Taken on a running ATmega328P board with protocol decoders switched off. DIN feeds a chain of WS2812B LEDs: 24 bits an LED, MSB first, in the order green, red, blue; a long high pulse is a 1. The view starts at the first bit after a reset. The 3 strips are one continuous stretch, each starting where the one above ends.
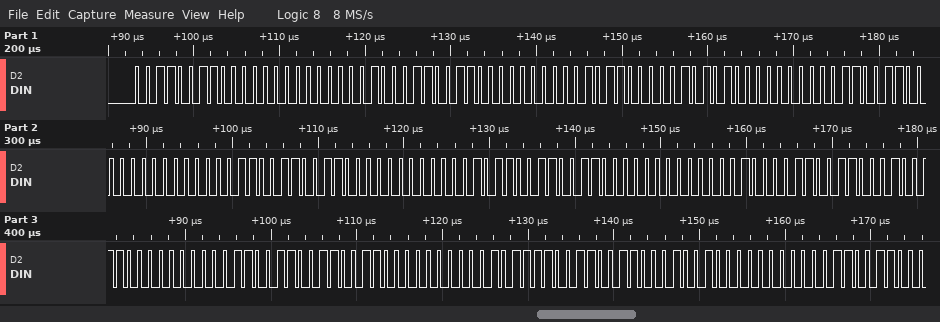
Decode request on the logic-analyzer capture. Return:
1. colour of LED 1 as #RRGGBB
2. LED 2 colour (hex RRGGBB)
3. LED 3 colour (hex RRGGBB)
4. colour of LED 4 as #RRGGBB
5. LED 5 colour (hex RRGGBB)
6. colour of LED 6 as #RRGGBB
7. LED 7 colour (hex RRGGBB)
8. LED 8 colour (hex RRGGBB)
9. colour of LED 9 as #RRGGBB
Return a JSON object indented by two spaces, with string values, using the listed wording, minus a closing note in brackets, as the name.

{
  "colour of LED 1 as #RRGGBB": "#003302",
  "LED 2 colour": "#00332C",
  "LED 3 colour": "#001533",
  "colour of LED 4 as #RRGGBB": "#030033",
  "LED 5 colour": "#0B0033",
  "colour of LED 6 as #RRGGBB": "#040033",
  "LED 7 colour": "#001333",
  "LED 8 colour": "#00332F",
  "colour of LED 9 as #RRGGBB": "#123300"
}
